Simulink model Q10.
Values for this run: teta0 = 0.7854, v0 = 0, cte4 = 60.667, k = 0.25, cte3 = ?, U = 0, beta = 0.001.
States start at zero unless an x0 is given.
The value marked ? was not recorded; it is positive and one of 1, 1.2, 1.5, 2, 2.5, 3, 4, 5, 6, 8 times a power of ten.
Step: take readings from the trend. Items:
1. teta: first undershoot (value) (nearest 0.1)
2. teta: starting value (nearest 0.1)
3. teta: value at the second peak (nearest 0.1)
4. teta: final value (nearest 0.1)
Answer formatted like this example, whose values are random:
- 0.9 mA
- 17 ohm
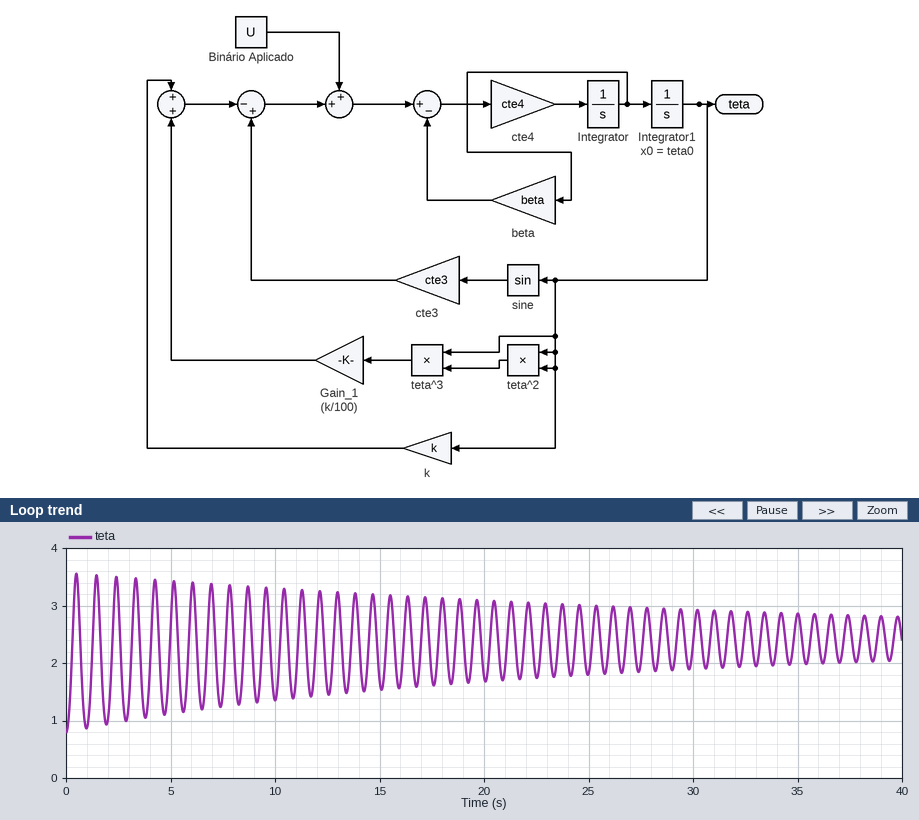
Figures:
- 0.9
- 0.8
- 3.5
- 2.4
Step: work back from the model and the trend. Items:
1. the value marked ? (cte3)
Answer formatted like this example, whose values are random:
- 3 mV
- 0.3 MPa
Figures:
- 1
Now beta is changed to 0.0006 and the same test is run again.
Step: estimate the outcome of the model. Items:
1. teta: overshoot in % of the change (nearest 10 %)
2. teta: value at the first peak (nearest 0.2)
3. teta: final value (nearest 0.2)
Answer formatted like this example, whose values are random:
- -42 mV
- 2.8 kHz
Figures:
- 70 %
- 3.6
- 2.4
